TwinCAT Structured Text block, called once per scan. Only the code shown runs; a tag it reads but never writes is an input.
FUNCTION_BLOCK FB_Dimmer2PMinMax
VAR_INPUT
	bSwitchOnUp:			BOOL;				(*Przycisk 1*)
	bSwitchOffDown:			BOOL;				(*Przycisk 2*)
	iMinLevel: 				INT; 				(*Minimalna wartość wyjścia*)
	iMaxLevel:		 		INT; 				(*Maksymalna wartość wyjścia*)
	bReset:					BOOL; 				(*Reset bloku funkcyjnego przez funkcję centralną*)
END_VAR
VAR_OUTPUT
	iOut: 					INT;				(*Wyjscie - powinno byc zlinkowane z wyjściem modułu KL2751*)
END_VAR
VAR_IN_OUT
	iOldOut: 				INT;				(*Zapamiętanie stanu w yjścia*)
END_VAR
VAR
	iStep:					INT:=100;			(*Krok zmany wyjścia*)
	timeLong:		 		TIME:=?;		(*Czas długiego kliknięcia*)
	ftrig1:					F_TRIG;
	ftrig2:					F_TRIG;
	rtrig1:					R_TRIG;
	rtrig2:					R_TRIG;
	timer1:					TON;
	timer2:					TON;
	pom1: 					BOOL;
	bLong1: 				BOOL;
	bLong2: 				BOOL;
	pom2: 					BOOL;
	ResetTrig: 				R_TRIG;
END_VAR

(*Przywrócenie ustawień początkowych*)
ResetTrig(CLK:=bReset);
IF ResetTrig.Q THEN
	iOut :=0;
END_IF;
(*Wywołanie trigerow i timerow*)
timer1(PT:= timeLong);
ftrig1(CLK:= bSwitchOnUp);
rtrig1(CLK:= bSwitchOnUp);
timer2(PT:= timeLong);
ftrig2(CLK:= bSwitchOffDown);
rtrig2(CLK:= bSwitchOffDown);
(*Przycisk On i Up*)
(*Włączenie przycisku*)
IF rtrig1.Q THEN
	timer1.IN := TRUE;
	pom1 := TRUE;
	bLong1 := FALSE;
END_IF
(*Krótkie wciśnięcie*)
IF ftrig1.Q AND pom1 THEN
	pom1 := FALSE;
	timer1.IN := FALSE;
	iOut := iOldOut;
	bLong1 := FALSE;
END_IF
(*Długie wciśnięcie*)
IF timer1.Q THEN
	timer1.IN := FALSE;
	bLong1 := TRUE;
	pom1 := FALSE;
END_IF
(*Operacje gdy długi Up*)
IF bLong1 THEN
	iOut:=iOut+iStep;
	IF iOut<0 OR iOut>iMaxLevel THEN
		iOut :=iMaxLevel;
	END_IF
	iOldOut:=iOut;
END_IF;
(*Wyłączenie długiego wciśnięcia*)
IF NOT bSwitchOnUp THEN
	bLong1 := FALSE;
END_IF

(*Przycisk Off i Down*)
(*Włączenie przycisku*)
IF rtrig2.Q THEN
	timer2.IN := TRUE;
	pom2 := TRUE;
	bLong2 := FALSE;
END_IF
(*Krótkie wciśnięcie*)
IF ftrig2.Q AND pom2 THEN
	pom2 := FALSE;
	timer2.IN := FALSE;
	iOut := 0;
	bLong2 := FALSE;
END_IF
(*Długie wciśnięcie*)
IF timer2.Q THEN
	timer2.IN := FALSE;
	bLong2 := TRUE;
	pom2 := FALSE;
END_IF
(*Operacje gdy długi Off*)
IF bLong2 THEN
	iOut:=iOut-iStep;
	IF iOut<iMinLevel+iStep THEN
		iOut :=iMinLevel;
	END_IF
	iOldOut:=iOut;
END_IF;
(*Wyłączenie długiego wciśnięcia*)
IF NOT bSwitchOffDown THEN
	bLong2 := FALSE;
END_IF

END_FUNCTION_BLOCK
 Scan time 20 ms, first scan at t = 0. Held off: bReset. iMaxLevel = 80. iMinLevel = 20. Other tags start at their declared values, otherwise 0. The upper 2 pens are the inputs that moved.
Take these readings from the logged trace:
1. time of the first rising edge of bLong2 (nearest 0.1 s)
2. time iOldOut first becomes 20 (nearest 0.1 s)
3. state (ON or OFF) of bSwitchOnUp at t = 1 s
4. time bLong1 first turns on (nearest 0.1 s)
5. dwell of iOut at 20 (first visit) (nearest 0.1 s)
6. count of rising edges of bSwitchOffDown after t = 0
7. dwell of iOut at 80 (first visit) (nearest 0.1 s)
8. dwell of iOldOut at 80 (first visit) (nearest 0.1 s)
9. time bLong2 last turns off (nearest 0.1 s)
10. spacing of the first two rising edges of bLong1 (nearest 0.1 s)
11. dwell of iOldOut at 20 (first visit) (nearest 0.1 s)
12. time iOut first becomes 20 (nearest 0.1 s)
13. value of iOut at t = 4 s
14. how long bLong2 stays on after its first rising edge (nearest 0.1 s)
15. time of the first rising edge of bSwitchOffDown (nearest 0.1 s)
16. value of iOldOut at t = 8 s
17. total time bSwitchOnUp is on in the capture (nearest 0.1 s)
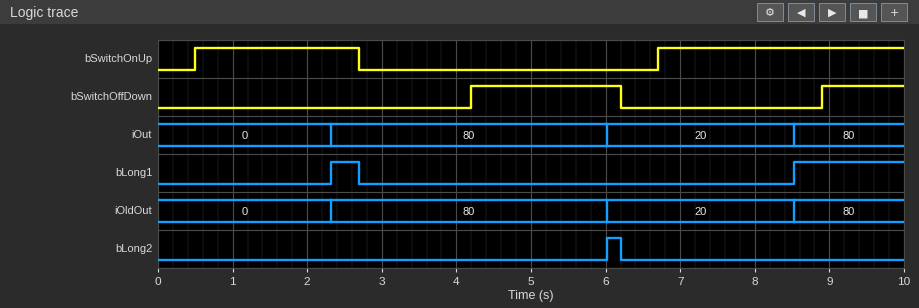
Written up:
6.0 s
6.0 s
ON
2.3 s
2.5 s
2
3.7 s
3.7 s
6.2 s
6.2 s
2.5 s
6.0 s
80
0.2 s
4.2 s
20
5.5 s
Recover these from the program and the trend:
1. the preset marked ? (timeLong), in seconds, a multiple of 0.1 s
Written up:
1.8 s
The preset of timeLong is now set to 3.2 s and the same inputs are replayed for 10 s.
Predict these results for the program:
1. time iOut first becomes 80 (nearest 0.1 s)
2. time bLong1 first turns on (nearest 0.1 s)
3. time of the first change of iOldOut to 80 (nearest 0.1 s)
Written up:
9.9 s
9.9 s
9.9 s
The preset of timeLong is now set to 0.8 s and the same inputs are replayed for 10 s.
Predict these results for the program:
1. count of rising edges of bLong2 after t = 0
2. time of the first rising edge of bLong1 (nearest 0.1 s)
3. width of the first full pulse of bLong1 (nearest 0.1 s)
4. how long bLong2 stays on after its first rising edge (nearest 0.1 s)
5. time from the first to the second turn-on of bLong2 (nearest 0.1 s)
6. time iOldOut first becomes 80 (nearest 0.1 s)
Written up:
2
1.3 s
1.4 s
1.2 s
4.7 s
1.3 s
